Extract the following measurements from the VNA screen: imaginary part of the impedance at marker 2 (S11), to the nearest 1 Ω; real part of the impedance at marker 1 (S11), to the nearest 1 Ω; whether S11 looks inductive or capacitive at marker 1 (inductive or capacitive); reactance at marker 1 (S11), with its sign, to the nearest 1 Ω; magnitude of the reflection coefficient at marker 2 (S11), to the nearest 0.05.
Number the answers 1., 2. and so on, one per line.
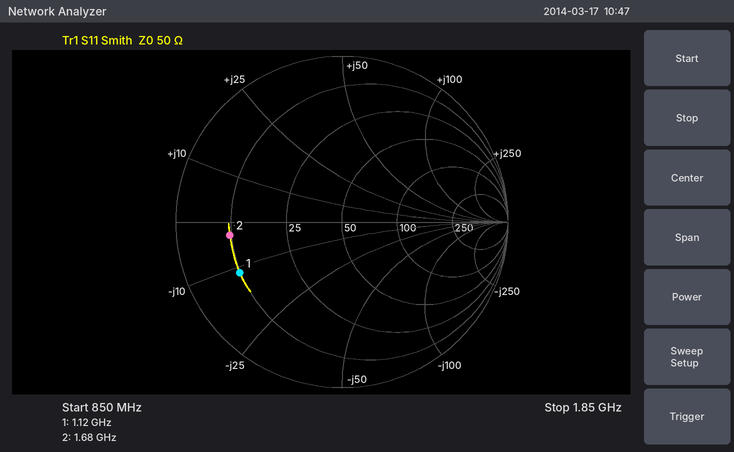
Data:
1. -3 Ω
2. 10 Ω
3. capacitive
4. -11 Ω
5. 0.70
